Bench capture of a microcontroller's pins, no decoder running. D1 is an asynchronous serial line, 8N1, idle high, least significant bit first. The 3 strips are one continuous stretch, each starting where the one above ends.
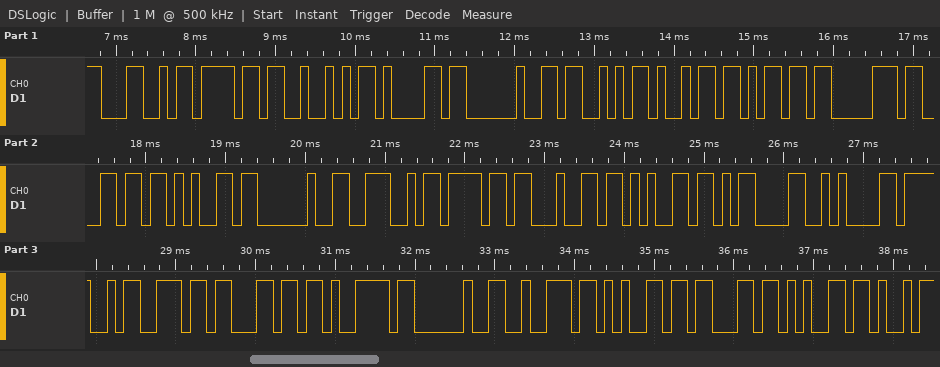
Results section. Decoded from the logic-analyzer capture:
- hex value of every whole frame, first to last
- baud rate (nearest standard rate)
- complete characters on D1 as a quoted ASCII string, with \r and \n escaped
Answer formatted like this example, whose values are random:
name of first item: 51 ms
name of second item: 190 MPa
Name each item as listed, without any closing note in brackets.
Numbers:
hex value of every whole frame, first to last: 0x4C 0x6F 0x52 0x61 0x20 0x53 0x69 0x6D 0x70 0x6C 0x65 0x20 0x4E 0x6F 0x64 0x65 0x0D 0x0A 0x4F 0x6E 0x6C 0x79 0x20 0x72 0x65 0x63 0x65
baud rate: 9600 baud
complete characters on D1 as a quoted ASCII string, with \r and \n escaped: "LoRa Simple Node\r\nOnly rece"
